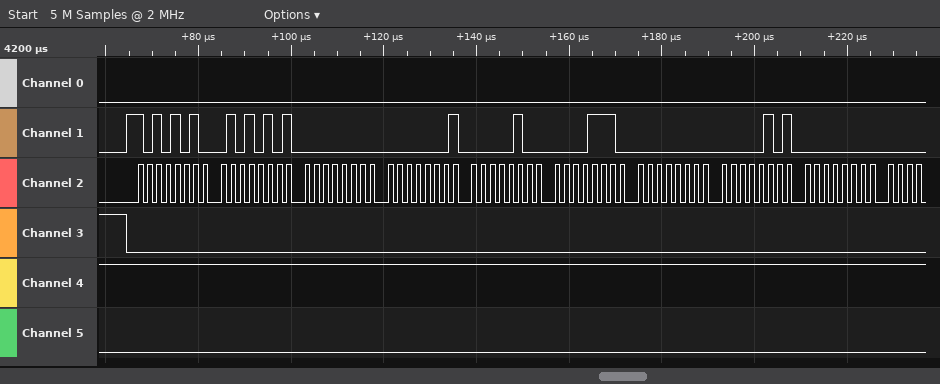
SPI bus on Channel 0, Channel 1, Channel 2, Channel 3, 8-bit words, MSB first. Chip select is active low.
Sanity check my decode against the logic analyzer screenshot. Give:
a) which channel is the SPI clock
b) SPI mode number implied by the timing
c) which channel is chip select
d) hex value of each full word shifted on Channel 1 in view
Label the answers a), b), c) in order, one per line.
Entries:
a) Channel 2
b) 0
c) Channel 3
d) AA, 55, 00, 01, 04, 0E, 00, 05, 00
